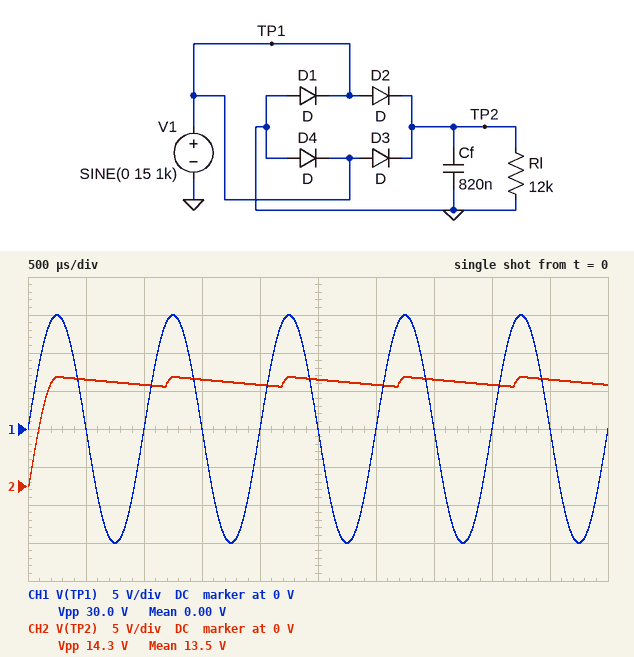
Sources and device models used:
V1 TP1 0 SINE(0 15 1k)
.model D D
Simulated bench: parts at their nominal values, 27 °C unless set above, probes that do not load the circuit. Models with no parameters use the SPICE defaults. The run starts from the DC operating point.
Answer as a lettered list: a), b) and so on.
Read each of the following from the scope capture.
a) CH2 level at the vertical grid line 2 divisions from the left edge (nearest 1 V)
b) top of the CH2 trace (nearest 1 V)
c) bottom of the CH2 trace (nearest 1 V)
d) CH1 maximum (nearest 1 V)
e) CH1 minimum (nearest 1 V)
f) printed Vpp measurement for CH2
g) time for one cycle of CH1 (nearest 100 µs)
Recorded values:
a) 13 V
b) 14 V
c) 0 V
d) 15 V
e) -15 V
f) 14.3 V
g) 1.0 ms
